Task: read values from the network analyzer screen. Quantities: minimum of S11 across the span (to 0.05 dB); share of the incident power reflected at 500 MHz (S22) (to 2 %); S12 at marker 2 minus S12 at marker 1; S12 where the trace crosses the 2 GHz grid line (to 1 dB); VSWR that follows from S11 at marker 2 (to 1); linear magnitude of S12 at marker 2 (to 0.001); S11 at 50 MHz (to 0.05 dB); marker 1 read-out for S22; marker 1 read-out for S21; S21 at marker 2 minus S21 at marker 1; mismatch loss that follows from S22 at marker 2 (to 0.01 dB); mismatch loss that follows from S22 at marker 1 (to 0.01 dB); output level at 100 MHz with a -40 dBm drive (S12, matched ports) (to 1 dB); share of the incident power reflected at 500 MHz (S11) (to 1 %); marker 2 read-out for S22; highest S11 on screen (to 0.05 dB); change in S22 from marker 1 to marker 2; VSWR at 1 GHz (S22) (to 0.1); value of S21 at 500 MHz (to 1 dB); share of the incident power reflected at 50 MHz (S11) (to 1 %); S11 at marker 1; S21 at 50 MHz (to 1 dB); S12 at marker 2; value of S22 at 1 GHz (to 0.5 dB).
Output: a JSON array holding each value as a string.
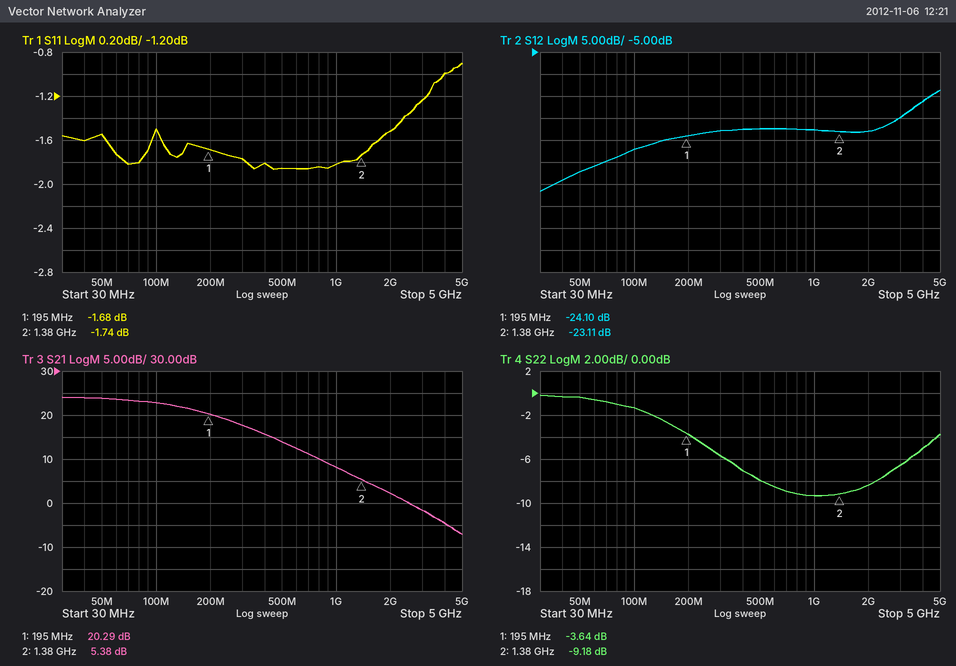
["-1.85 dB", "16 %", "0.99 dB", "-23 dB", "10", "0.070", "-1.55 dB", "-3.64 dB", "20.29 dB", "-14.91 dB", "0.56 dB", "2.46 dB", "-67 dBm", "65 %", "-9.18 dB", "-0.90 dB", "-5.54 dB", "2.0", "14 dB", "70 %", "-1.68 dB", "24 dB", "-23.11 dB", "-9.5 dB"]
